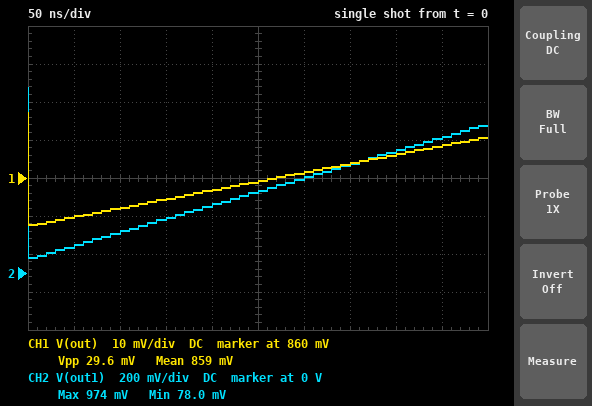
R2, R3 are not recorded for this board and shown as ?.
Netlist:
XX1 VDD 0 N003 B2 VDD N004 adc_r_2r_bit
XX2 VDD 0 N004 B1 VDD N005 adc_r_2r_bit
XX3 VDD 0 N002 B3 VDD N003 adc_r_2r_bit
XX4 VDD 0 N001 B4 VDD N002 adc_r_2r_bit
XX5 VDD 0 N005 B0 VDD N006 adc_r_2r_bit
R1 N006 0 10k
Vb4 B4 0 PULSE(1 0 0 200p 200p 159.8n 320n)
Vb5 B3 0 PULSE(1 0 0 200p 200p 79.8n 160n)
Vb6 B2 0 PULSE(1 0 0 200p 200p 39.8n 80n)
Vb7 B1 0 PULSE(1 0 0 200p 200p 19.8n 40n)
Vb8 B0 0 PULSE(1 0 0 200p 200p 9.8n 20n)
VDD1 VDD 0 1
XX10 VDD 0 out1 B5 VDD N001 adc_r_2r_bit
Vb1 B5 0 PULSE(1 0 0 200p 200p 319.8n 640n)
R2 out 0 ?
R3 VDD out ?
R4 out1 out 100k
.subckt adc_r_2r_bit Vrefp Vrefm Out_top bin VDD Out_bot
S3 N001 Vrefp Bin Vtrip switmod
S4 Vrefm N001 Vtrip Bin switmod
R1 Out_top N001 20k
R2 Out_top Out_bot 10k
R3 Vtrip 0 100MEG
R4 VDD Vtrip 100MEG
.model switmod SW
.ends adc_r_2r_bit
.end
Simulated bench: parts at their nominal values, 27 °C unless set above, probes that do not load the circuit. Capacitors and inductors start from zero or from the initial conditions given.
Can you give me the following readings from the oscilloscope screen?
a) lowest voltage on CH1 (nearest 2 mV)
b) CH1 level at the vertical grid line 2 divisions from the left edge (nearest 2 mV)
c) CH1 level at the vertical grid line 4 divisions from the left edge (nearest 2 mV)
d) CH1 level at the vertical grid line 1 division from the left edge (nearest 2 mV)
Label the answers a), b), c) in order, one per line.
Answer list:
a) 848 mV
b) 852 mV
c) 856 mV
d) 850 mV
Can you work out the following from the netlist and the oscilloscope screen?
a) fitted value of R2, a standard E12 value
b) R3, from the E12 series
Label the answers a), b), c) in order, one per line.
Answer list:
a) 27 kΩ
b) 3.9 kΩ
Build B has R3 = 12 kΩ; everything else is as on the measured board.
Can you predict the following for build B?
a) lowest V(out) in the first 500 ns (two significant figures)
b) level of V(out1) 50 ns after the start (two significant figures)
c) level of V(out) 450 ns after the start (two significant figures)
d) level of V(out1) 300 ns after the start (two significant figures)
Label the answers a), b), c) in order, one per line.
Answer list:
a) 640 mV
b) 120 mV
c) 690 mV
d) 470 mV
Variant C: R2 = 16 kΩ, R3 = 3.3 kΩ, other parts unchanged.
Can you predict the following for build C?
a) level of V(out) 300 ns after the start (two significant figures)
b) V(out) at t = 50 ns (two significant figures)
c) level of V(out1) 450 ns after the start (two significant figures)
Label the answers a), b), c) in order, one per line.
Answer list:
a) 820 mV
b) 810 mV
c) 700 mV
